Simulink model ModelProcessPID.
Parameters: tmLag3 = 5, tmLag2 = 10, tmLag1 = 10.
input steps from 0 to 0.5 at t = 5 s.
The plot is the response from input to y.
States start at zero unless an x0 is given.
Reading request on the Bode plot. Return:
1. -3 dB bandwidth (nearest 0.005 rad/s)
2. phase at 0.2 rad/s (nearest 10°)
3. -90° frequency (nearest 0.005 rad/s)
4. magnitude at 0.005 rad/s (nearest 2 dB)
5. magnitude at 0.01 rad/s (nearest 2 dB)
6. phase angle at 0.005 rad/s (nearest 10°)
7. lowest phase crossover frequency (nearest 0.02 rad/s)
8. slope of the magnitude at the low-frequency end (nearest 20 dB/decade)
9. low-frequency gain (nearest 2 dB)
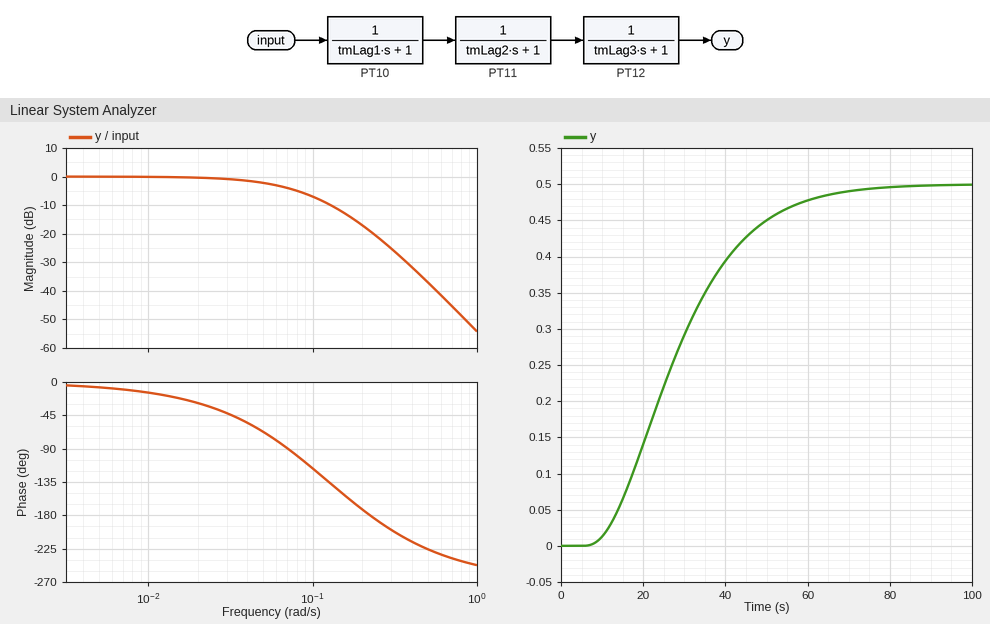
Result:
0.060 rad/s
-170°
0.070 rad/s
0 dB
0 dB
-10°
0.22 rad/s
0 dB/decade
0 dB
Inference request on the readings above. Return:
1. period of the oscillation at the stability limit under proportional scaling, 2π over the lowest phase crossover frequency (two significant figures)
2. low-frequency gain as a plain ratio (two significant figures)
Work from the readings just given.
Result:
29 s
1.0
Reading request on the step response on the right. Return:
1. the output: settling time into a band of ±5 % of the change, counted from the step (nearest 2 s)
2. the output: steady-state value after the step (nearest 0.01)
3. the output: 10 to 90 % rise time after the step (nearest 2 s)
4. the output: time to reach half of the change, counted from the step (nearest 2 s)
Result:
54 s
0.50
36 s
22 s
